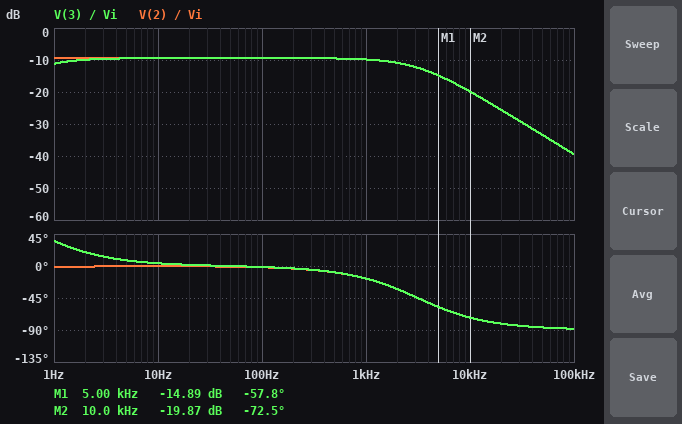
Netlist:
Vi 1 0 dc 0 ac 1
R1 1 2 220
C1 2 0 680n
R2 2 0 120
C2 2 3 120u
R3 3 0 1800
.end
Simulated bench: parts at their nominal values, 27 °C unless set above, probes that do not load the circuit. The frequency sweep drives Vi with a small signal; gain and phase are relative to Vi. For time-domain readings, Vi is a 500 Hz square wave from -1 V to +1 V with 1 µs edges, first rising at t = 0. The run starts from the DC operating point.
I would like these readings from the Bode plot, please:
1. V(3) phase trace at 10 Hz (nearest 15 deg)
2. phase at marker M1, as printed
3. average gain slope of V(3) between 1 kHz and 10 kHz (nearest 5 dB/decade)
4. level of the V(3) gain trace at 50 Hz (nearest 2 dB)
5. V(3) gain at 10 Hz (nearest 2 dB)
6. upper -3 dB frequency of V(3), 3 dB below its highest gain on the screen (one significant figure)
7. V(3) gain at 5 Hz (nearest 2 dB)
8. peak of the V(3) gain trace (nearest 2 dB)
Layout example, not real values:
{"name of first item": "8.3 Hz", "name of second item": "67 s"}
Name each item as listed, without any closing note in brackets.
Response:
{"V(3) phase trace at 10 Hz": "0 deg", "phase at marker M1, as printed": "-57.8 deg", "average gain slope of V(3) between 1 kHz and 10 kHz": "-10 dB/decade", "level of the V(3) gain trace at 50 Hz": "-10 dB", "V(3) gain at 10 Hz": "-10 dB", "upper -3 dB frequency of V(3), 3 dB below its highest gain on the screen": "3 kHz", "V(3) gain at 5 Hz": "-10 dB", "peak of the V(3) gain trace": "-10 dB"}
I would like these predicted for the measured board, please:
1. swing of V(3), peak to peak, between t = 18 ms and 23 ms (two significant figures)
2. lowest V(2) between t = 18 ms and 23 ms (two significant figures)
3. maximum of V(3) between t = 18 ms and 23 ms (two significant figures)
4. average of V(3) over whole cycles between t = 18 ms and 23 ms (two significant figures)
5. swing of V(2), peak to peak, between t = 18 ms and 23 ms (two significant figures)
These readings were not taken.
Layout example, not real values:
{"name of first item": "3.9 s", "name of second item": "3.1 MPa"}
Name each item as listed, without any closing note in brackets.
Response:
{"swing of V(3), peak to peak, between t = 18 ms and 23 ms": "680 mV", "lowest V(2) between t = 18 ms and 23 ms": "-350 mV", "maximum of V(3) between t = 18 ms and 23 ms": "650 mV", "average of V(3) over whole cycles between t = 18 ms and 23 ms": "310 mV", "swing of V(2), peak to peak, between t = 18 ms and 23 ms": "680 mV"}
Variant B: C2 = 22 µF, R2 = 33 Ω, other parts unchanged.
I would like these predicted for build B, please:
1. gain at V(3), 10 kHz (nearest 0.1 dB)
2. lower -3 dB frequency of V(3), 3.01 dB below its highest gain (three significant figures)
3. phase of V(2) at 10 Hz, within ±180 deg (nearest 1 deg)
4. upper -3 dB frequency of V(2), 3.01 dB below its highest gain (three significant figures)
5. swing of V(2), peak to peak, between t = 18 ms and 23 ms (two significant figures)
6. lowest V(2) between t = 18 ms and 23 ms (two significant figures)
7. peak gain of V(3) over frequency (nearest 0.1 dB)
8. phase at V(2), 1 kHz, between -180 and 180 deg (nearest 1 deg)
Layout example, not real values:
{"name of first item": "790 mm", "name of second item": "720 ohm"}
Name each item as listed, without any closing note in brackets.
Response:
{"gain at V(3), 10 kHz": "-21.7 dB", "lower -3 dB frequency of V(3), 3.01 dB below its highest gain": "3.95 Hz", "phase of V(2) at 10 Hz, within ±180 deg": "0 deg", "upper -3 dB frequency of V(2), 3.01 dB below its highest gain": "8.02 kHz", "swing of V(2), peak to peak, between t = 18 ms and 23 ms": "260 mV", "lowest V(2) between t = 18 ms and 23 ms": "-130 mV", "peak gain of V(3) over frequency": "-17.8 dB", "phase at V(2), 1 kHz, between -180 and 180 deg": "-7 deg"}
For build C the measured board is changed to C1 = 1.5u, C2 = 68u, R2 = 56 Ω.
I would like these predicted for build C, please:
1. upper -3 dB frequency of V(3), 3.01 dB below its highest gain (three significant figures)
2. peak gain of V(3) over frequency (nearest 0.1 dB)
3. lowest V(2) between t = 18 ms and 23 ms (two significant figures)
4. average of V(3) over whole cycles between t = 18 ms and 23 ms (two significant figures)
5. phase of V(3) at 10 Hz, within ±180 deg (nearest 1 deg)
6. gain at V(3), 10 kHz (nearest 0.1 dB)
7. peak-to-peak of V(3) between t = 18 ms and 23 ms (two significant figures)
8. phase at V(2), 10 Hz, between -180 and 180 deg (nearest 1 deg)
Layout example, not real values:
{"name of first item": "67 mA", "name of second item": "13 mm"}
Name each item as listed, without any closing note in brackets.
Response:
{"upper -3 dB frequency of V(3), 3.01 dB below its highest gain": "2.44 kHz", "peak gain of V(3) over frequency": "-14.1 dB", "lowest V(2) between t = 18 ms and 23 ms": "-200 mV", "average of V(3) over whole cycles between t = 18 ms and 23 ms": "170 mV", "phase of V(3) at 10 Hz, within ±180 deg": "7 deg", "gain at V(3), 10 kHz": "-26.6 dB", "peak-to-peak of V(3) between t = 18 ms and 23 ms": "400 mV", "phase at V(2), 10 Hz, between -180 and 180 deg": "0 deg"}
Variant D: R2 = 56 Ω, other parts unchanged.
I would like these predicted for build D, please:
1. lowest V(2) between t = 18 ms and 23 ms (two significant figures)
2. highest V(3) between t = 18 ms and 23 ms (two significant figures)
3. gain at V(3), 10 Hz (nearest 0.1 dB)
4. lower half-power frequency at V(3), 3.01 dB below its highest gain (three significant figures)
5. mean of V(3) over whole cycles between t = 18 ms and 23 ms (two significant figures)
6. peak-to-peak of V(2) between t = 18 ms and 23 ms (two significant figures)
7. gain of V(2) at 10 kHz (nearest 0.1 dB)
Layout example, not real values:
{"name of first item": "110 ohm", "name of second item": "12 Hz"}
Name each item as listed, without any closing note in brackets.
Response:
{"lowest V(2) between t = 18 ms and 23 ms": "-200 mV", "highest V(3) between t = 18 ms and 23 ms": "380 mV", "gain at V(3), 10 Hz": "-14.1 dB", "lower half-power frequency at V(3), 3.01 dB below its highest gain": "719 mHz", "mean of V(3) over whole cycles between t = 18 ms and 23 ms": "180 mV", "peak-to-peak of V(2) between t = 18 ms and 23 ms": "400 mV", "gain of V(2) at 10 kHz": "-20.6 dB"}
